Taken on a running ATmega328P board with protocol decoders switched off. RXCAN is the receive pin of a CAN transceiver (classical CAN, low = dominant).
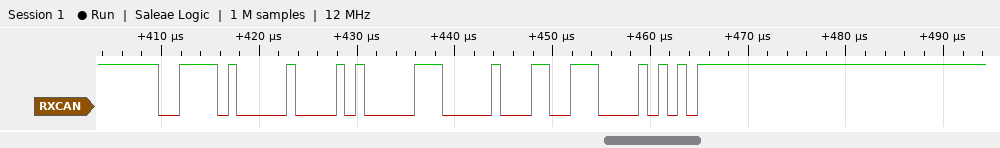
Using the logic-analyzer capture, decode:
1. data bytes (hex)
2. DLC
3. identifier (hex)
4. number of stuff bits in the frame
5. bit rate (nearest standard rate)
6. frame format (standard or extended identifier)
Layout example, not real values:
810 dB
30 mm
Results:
83 00
2
0x3D0
3
1000 kbit/s
standard
